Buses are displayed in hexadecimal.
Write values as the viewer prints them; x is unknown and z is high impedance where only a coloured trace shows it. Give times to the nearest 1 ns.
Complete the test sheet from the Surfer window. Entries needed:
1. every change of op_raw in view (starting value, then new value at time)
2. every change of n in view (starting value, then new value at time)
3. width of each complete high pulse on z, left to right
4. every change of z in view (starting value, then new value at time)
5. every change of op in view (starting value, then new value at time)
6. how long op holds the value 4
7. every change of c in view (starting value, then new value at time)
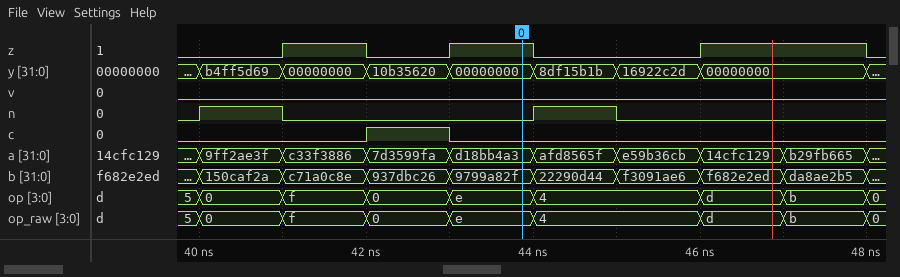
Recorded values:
5, 0 at 40 ns, f at 41 ns, 0 at 42 ns, e at 43 ns, 4 at 44 ns, d at 46 ns, b at 47 ns, 0 at 48 ns
0, 1 at 40 ns, 0 at 41 ns, 1 at 44 ns, 0 at 45 ns
1 ns, 1 ns, 2 ns
0, 1 at 41 ns, 0 at 42 ns, 1 at 43 ns, 0 at 44 ns, 1 at 46 ns, 0 at 48 ns
5, 0 at 40 ns, f at 41 ns, 0 at 42 ns, e at 43 ns, 4 at 44 ns, d at 46 ns, b at 47 ns, 0 at 48 ns
2 ns
0, 1 at 42 ns, 0 at 43 ns
